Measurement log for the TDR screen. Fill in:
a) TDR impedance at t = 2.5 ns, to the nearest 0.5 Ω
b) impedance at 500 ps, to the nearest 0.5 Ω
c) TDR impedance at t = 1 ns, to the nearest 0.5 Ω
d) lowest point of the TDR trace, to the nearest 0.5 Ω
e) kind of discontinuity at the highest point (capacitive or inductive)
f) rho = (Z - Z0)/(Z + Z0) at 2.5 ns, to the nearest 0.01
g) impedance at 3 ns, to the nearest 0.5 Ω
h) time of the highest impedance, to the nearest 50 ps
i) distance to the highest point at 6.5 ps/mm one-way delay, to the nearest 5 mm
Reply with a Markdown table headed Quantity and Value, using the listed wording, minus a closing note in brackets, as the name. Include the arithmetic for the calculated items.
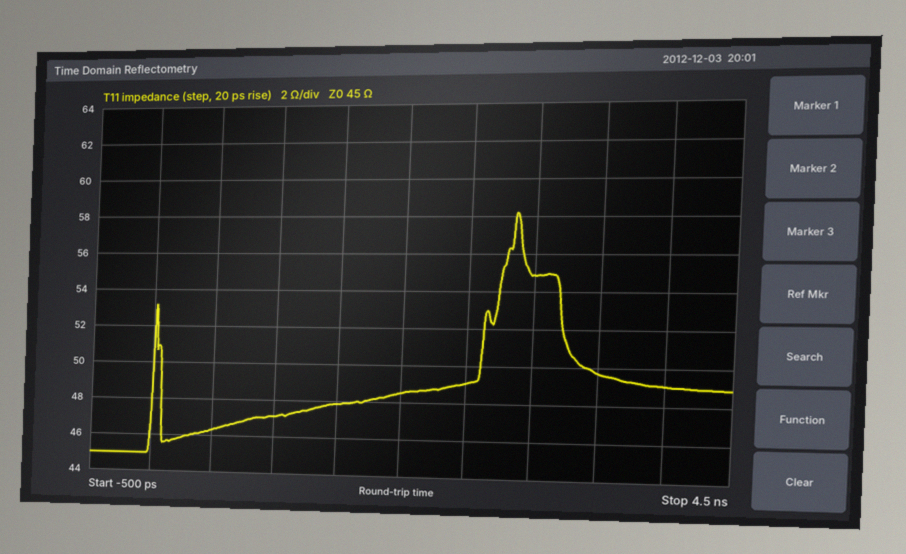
| Quantity | Value |
|---|---|
| TDR impedance at t = 2.5 ns, to the nearest 0.5 Ω | 49.0 Ω |
| impedance at 500 ps, to the nearest 0.5 Ω | 46.5 Ω |
| TDR impedance at t = 1 ns, to the nearest 0.5 Ω | 47.0 Ω |
| lowest point of the TDR trace, to the nearest 0.5 Ω | 45.0 Ω |
| kind of discontinuity at the highest point | inductive |
| rho = (Z - Z0)/(Z + Z0) at 2.5 ns, to the nearest 0.01 | (49 − 45)/(49 + 45) ≈ +0.04 |
| impedance at 3 ns, to the nearest 0.5 Ω | 55.0 Ω |
| time of the highest impedance, to the nearest 50 ps | 2.85 ns |
| distance to the highest point at 6.5 ps/mm one-way delay, to the nearest 5 mm | 2.85 ns / 2 / 6.5 ps/mm ≈ 219 mm, so 220 mm to the nearest 5 mm |
